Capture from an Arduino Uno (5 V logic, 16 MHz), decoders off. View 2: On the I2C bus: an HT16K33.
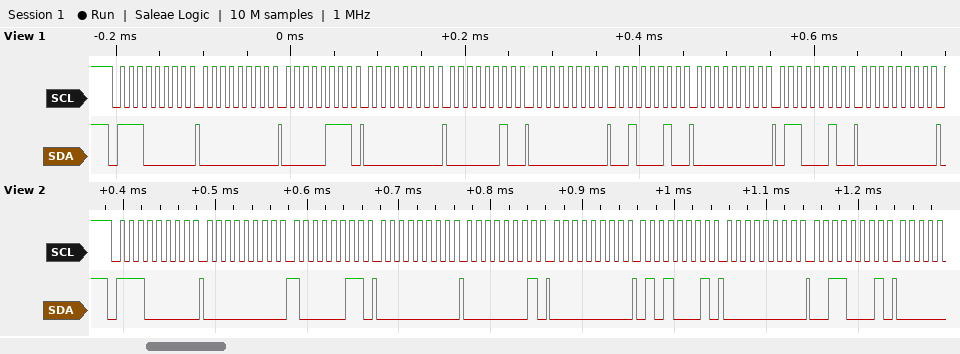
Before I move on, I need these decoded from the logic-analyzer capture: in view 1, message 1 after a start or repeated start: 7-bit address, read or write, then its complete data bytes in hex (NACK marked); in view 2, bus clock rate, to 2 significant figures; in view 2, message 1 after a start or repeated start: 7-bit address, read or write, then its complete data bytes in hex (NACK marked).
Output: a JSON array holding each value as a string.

["0x70 write: 00 07 00 02 00 22 00 62 00", "100 kHz", "0x70 write: 00 83 00 01 00 51 00 31"]
